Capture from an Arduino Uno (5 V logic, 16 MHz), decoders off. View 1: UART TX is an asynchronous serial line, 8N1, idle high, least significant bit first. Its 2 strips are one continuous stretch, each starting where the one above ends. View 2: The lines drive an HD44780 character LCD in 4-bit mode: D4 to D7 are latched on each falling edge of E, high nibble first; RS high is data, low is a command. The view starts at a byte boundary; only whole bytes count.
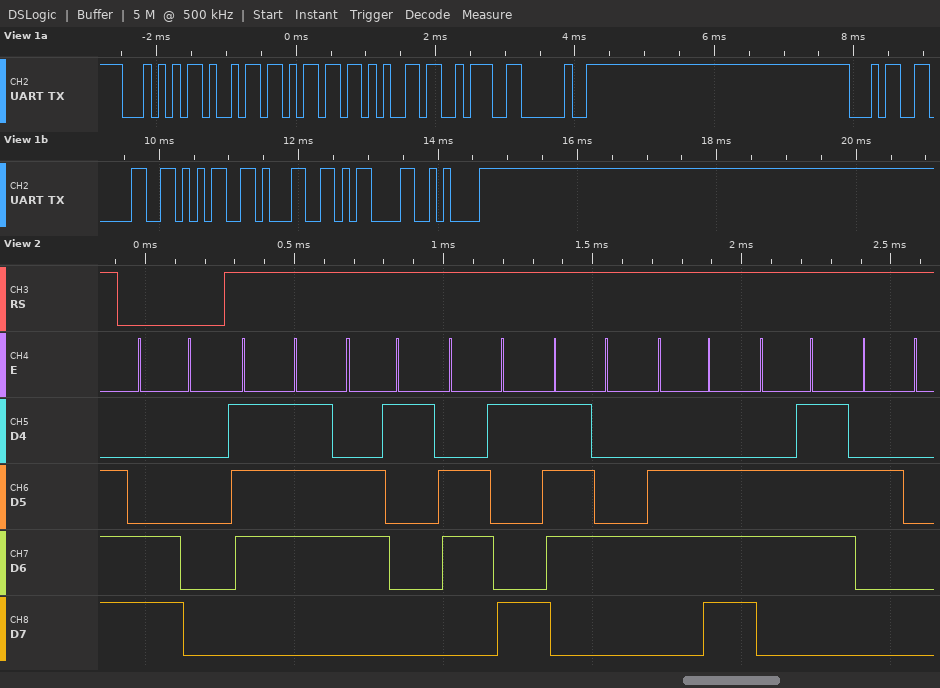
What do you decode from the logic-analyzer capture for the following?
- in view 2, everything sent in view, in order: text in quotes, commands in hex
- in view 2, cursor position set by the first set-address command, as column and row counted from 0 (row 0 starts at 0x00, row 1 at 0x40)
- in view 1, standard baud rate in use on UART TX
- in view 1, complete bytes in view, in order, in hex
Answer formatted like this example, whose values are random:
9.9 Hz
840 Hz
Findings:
0xC0 "waitng "
column 0, row 1
9600 baud
54 69 6D 65 3A 20 34 30 35 31 0D 0A
